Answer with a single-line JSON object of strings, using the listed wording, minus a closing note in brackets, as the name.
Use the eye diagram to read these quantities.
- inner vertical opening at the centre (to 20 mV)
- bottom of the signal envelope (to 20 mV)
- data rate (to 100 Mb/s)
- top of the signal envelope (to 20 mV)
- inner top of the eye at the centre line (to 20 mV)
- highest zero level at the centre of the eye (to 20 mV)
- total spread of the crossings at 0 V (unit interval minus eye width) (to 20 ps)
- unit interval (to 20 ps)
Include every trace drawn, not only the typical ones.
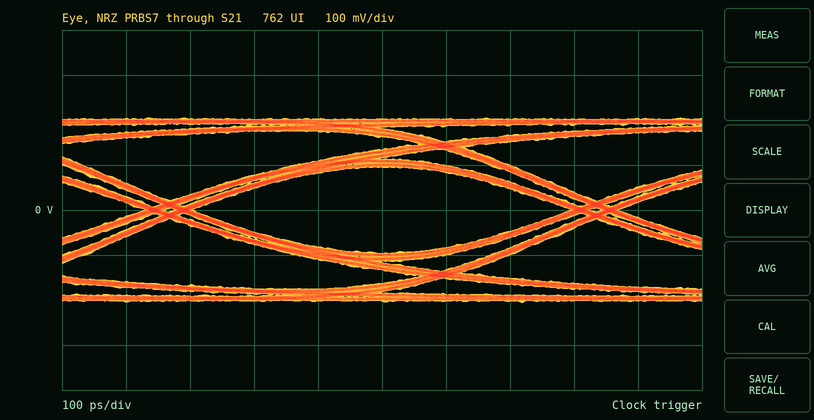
{"inner vertical opening at the centre": "200 mV", "bottom of the signal envelope": "-200 mV", "data rate": "1.5 Gb/s", "top of the signal envelope": "200 mV", "inner top of the eye at the centre line": "100 mV", "highest zero level at the centre of the eye": "-100 mV", "total spread of the crossings at 0 V (unit interval minus eye width)": "80 ps", "unit interval": "660 ps"}
